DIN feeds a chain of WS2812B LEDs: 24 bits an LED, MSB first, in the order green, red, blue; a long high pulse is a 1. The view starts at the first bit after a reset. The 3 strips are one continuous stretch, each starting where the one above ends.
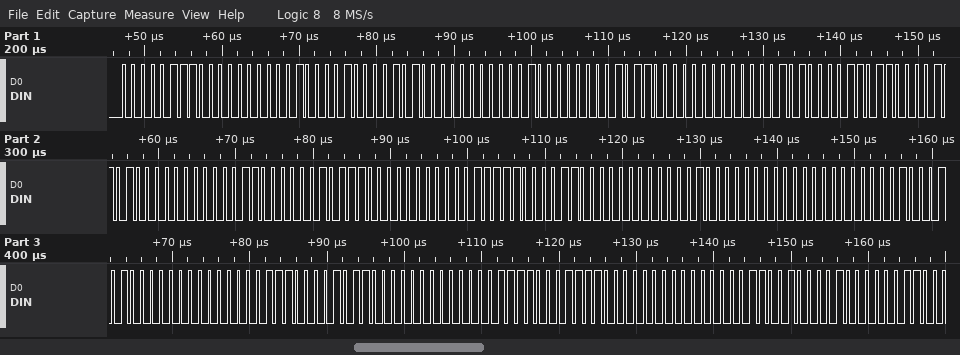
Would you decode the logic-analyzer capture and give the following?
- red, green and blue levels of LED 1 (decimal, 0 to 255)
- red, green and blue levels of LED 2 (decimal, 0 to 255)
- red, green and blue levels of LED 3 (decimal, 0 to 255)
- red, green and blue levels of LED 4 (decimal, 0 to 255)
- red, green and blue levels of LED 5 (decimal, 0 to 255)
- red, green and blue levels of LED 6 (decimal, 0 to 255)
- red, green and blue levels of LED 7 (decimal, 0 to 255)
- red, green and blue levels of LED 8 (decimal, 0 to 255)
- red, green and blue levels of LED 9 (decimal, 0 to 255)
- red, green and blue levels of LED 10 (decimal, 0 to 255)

0, 7, 33
0, 10, 32
0, 22, 10
13, 27, 0
23, 24, 0
12, 31, 0
0, 32, 1
0, 20, 14
0, 22, 15
0, 30, 3
